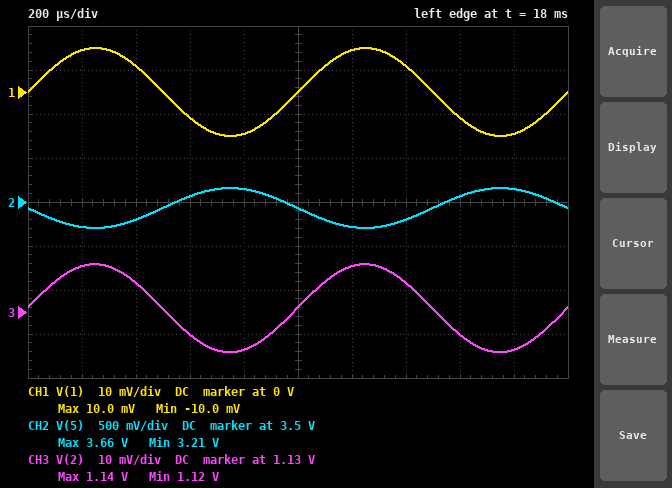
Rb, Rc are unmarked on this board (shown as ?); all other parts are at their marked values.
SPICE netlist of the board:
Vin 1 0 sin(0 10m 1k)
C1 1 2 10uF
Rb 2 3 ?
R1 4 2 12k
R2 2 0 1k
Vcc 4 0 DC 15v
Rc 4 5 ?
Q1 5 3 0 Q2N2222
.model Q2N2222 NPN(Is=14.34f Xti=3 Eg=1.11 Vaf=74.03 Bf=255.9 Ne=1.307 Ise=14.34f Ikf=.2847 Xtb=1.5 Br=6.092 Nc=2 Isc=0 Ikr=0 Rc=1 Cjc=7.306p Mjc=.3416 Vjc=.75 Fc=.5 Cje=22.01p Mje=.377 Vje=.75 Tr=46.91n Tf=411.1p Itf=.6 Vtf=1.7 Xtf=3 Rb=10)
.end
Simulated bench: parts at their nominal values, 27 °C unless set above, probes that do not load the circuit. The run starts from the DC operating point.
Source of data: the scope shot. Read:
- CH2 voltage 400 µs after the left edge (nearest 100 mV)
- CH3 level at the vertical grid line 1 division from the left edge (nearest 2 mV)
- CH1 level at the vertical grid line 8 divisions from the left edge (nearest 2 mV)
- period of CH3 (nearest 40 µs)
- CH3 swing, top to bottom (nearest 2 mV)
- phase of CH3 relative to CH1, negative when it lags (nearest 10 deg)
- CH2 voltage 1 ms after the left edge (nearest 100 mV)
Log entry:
3.3 V
1.140 V
-6 mV
1.00 ms
20 mV
0 deg
3.4 V
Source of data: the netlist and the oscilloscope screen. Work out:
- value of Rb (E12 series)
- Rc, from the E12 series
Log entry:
18 kΩ
2.7 kΩ
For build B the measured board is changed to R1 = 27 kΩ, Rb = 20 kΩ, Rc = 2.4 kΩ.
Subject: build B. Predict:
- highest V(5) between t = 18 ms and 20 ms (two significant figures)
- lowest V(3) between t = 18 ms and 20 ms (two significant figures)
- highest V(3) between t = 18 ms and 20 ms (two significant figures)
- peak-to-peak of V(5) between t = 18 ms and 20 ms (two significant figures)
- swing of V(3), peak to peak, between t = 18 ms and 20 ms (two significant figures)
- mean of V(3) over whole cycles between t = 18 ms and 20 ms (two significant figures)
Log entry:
15 V
520 mV
540 mV
26 mV
18 mV
530 mV
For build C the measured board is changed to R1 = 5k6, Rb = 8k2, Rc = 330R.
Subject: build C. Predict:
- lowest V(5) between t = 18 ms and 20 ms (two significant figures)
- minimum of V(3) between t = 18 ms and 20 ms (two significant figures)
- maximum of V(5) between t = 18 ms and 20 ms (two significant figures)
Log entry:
4.6 V
740 mV
4.7 V
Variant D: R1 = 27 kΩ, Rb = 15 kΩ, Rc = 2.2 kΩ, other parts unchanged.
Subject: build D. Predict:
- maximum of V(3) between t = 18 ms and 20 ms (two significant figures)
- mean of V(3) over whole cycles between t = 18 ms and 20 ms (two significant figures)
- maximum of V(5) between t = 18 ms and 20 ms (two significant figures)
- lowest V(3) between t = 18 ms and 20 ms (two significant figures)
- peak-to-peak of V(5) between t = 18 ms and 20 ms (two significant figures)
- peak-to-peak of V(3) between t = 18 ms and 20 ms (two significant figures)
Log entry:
540 mV
530 mV
15 V
520 mV
25 mV
19 mV
